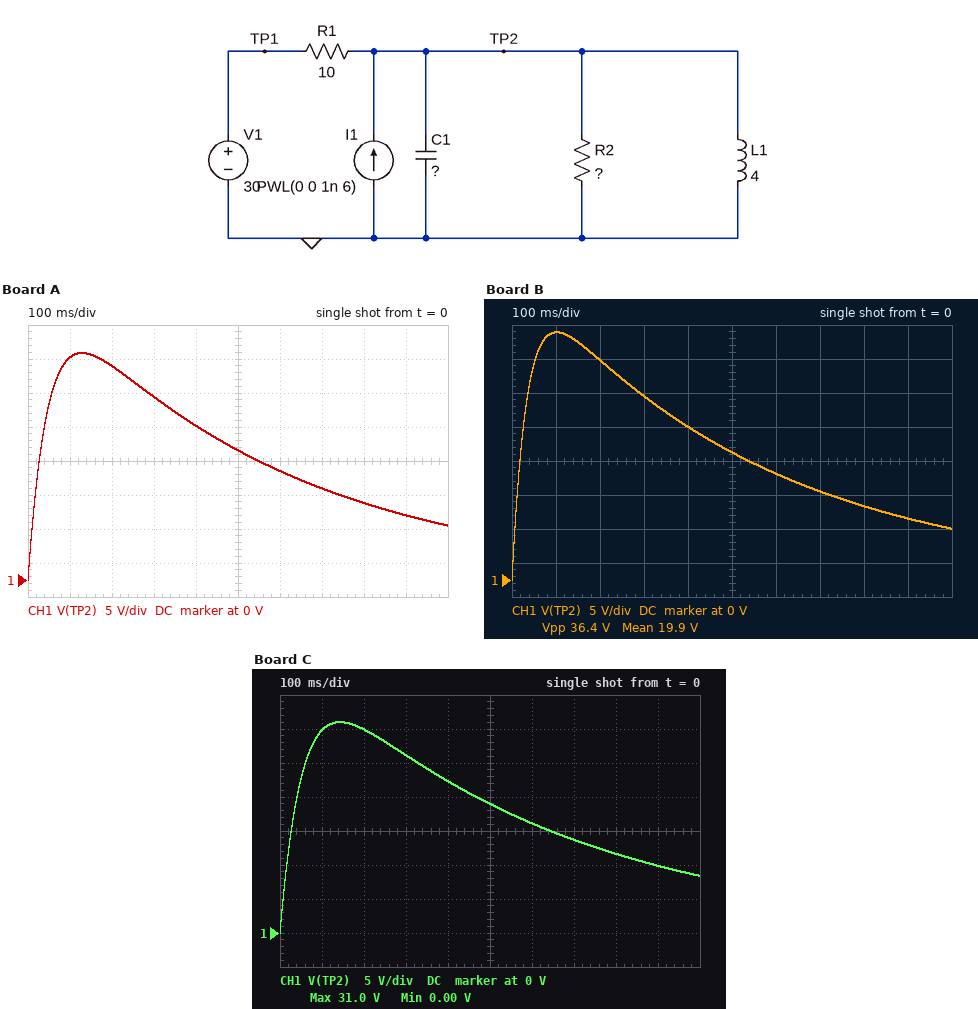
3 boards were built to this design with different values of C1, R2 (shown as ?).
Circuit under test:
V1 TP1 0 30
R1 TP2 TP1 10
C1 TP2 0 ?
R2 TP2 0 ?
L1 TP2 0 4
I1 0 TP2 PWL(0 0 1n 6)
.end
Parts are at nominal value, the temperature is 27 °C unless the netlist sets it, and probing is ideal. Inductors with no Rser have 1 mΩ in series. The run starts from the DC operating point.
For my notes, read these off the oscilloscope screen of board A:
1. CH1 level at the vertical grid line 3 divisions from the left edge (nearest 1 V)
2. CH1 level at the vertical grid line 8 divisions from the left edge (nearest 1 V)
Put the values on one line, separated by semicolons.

27 V; 11 V
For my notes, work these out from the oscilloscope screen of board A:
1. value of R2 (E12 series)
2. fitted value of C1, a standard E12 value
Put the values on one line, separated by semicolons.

18 Ω; 6.8 mF
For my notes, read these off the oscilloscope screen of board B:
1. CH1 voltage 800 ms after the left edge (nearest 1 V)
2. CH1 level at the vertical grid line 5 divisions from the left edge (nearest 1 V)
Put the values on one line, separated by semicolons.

11 V; 19 V
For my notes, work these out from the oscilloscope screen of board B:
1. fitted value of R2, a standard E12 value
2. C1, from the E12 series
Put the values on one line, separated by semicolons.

22 Ω; 4.7 mF
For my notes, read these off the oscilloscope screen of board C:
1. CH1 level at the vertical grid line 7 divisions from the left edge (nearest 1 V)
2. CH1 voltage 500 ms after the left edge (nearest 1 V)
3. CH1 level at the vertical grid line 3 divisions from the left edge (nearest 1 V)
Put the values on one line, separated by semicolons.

14 V; 19 V; 26 V
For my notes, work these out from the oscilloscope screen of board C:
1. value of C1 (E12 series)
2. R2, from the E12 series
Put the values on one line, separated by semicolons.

8.2 mF; 15 Ω
